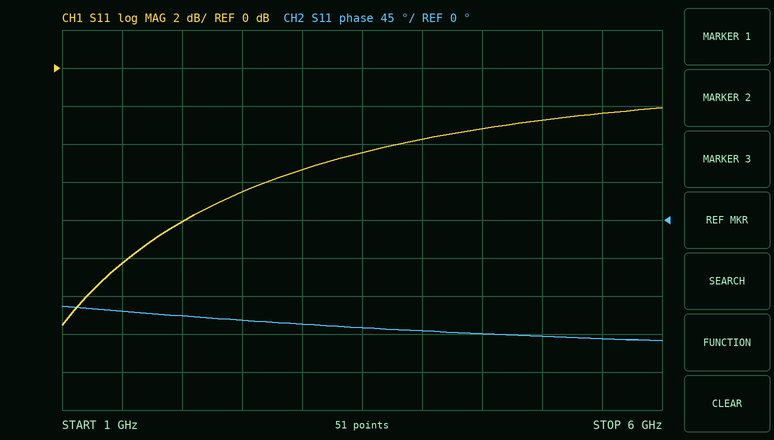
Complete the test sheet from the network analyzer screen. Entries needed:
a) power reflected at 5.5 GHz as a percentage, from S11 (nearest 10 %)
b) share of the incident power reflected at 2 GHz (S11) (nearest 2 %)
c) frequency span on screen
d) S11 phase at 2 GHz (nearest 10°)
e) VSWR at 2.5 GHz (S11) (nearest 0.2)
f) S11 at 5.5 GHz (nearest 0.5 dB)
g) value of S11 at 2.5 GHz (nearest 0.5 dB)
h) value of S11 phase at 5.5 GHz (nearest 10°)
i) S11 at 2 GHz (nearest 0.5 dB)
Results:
60 %
16 %
5 GHz
-110°
2.8
-2.5 dB
-6.5 dB
-140°
-8.0 dB
